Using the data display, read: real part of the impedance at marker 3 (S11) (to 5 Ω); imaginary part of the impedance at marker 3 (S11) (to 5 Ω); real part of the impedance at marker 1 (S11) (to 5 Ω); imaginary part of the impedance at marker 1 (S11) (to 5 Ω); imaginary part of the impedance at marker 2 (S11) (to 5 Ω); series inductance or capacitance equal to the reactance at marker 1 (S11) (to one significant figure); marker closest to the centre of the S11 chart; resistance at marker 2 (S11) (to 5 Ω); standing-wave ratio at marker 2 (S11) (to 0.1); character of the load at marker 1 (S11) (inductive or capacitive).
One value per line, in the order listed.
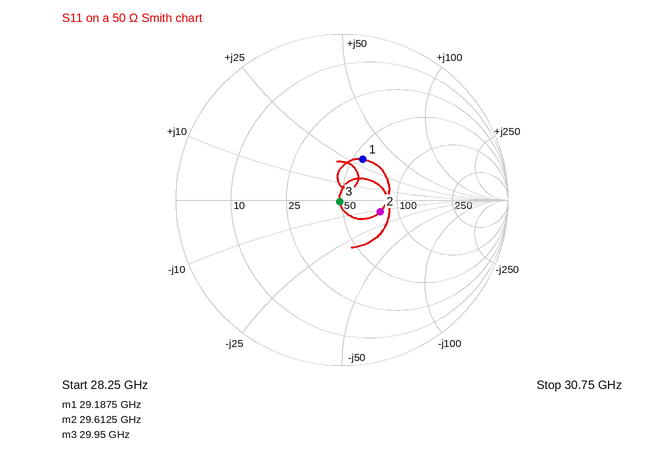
50 Ω
0 Ω
55 Ω
+30 Ω
-10 Ω
200 pH
marker 3
80 Ω
1.6
inductive
